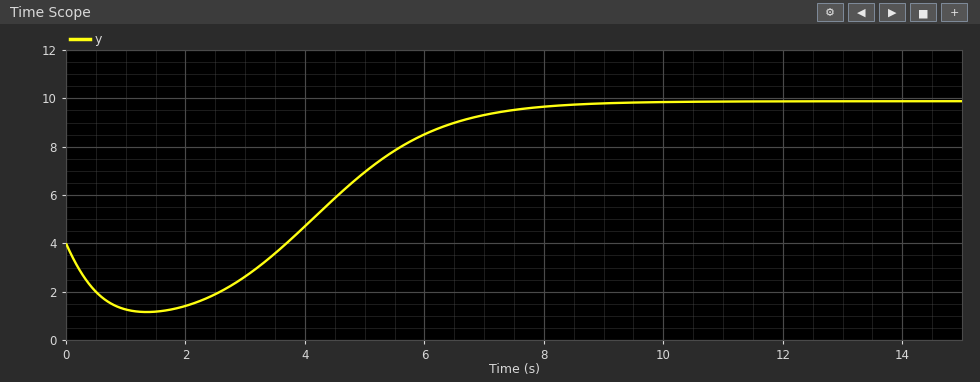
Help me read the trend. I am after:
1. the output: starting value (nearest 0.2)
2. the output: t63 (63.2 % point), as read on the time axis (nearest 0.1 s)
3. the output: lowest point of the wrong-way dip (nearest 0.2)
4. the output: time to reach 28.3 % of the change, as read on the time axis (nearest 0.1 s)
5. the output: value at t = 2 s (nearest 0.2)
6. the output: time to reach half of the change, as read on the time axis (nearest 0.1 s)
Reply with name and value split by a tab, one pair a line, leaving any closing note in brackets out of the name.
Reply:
the output: starting value	4.0
the output: t63 (63.2 % point), as read on the time axis	5.4 s
the output: lowest point of the wrong-way dip	1.2
the output: time to reach 28.3 % of the change, as read on the time axis	4.4 s
the output: value at t = 2 s	1.4
the output: time to reach half of the change, as read on the time axis	5.0 s
